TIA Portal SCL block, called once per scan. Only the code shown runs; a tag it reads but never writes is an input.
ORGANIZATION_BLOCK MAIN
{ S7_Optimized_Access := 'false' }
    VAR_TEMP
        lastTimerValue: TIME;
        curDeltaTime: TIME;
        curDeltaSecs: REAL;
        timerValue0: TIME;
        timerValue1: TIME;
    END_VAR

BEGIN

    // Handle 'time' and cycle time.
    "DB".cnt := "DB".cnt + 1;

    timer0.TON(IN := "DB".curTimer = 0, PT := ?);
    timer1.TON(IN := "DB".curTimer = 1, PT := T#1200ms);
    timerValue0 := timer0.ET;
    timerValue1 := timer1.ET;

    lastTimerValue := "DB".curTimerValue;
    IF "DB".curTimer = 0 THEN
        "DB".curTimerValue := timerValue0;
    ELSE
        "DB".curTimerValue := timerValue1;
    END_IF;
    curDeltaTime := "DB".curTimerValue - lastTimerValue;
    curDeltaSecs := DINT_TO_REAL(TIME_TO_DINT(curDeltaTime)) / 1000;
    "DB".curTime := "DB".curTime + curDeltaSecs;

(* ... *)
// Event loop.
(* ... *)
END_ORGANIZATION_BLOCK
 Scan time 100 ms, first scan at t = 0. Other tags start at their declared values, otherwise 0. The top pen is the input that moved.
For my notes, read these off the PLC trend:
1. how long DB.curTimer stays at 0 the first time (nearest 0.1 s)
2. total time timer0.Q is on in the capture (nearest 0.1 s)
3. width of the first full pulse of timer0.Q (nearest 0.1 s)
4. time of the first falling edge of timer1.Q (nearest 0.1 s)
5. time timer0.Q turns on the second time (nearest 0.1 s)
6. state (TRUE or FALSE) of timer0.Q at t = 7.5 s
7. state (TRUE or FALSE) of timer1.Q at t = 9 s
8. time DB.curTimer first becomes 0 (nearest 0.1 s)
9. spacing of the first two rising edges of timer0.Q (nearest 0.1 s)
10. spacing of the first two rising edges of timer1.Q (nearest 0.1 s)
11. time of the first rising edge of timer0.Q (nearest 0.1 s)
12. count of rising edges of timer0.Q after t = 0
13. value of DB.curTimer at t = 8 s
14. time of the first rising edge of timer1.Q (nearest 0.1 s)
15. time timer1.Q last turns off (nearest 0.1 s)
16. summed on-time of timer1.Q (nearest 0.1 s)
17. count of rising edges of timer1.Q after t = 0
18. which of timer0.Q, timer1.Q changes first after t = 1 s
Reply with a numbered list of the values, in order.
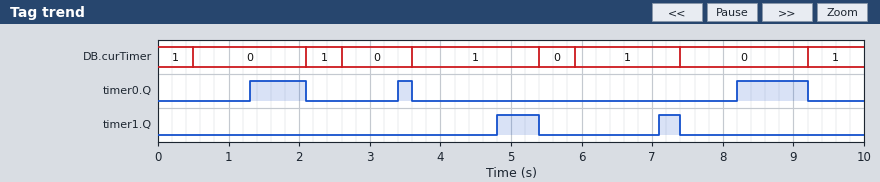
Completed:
1. 1.6 s
2. 2.0 s
3. 0.8 s
4. 5.4 s
5. 3.4 s
6. FALSE
7. FALSE
8. 0.5 s
9. 2.1 s
10. 2.3 s
11. 1.3 s
12. 3
13. 0
14. 4.8 s
15. 7.4 s
16. 0.9 s
17. 2
18. timer0.Q
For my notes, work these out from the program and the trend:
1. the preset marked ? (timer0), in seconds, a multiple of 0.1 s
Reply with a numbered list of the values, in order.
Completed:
1. 0.8 s
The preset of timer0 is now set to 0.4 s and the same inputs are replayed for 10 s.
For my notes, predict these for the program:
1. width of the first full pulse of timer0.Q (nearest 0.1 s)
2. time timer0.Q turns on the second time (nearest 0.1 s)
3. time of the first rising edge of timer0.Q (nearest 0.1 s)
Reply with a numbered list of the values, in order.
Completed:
1. 1.2 s
2. 3.0 s
3. 0.9 s
